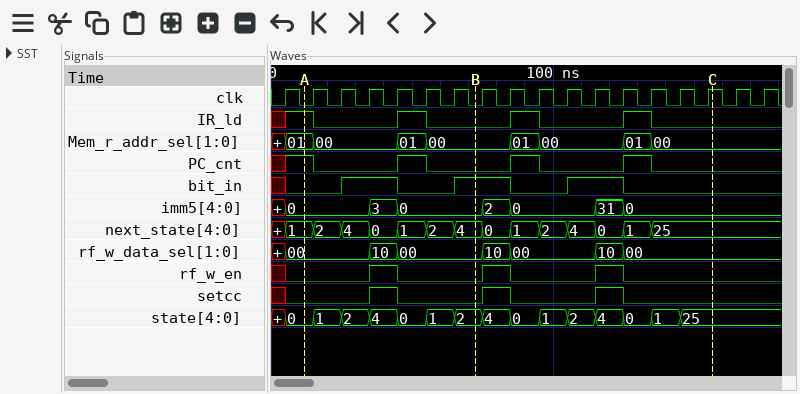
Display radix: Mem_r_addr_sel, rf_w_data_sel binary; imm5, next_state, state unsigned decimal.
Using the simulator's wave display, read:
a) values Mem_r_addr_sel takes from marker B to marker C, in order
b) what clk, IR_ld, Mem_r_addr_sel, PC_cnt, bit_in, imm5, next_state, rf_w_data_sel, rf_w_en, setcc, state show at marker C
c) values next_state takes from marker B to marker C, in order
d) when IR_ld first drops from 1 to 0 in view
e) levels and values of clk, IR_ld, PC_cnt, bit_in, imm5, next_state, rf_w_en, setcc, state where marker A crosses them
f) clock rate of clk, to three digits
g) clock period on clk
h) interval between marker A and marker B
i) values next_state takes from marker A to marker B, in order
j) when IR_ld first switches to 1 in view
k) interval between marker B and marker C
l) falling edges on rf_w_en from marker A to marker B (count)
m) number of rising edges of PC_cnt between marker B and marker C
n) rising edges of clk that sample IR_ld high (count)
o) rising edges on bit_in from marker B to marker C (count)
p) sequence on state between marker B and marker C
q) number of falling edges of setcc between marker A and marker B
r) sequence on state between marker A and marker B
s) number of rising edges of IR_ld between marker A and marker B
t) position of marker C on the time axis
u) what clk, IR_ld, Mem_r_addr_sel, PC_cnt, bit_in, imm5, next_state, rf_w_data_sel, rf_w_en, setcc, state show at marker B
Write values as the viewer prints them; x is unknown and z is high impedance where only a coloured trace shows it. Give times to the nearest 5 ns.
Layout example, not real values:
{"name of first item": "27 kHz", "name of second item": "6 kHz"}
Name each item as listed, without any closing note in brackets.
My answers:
{"values Mem_r_addr_sel takes from marker B to marker C, in order": "00, 01, 00, 01, 00", "what clk, IR_ld, Mem_r_addr_sel, PC_cnt, bit_in, imm5, next_state, rf_w_data_sel, rf_w_en, setcc, state show at marker C": "clk=1, IR_ld=0, Mem_r_addr_sel=00, PC_cnt=0, bit_in=0, imm5=0, next_state=25, rf_w_data_sel=00, rf_w_en=0, setcc=0, state=25", "values next_state takes from marker B to marker C, in order": "4, 0, 1, 2, 4, 0, 1, 25", "when IR_ld first drops from 1 to 0 in view": "15 ns", "levels and values of clk, IR_ld, PC_cnt, bit_in, imm5, next_state, rf_w_en, setcc, state where marker A crosses them": "clk=0, IR_ld=1, PC_cnt=1, bit_in=0, imm5=0, next_state=1, rf_w_en=0, setcc=0, state=0", "clock rate of clk, to three digits": "100 MHz", "clock period on clk": "10 ns", "interval between marker A and marker B": "60 ns", "values next_state takes from marker A to marker B, in order": "1, 2, 4, 0, 1, 2, 4", "when IR_ld first switches to 1 in view": "5 ns", "interval between marker B and marker C": "85 ns", "falling edges on rf_w_en from marker A to marker B": "1", "number of rising edges of PC_cnt between marker B and marker C": "2", "rising edges of clk that sample IR_ld high": "4", "rising edges on bit_in from marker B to marker C": "1", "sequence on state between marker B and marker C": "2, 4, 0, 1, 2, 4, 0, 1, 25", "number of falling edges of setcc between marker A and marker B": "1", "sequence on state between marker A and marker B": "0, 1, 2, 4, 0, 1, 2", "number of rising edges of IR_ld between marker A and marker B": "1", "position of marker C on the time axis": "155 ns", "what clk, IR_ld, Mem_r_addr_sel, PC_cnt, bit_in, imm5, next_state, rf_w_data_sel, rf_w_en, setcc, state show at marker B": "clk=0, IR_ld=0, Mem_r_addr_sel=00, PC_cnt=0, bit_in=1, imm5=0, next_state=4, rf_w_data_sel=00, rf_w_en=0, setcc=0, state=2"}
